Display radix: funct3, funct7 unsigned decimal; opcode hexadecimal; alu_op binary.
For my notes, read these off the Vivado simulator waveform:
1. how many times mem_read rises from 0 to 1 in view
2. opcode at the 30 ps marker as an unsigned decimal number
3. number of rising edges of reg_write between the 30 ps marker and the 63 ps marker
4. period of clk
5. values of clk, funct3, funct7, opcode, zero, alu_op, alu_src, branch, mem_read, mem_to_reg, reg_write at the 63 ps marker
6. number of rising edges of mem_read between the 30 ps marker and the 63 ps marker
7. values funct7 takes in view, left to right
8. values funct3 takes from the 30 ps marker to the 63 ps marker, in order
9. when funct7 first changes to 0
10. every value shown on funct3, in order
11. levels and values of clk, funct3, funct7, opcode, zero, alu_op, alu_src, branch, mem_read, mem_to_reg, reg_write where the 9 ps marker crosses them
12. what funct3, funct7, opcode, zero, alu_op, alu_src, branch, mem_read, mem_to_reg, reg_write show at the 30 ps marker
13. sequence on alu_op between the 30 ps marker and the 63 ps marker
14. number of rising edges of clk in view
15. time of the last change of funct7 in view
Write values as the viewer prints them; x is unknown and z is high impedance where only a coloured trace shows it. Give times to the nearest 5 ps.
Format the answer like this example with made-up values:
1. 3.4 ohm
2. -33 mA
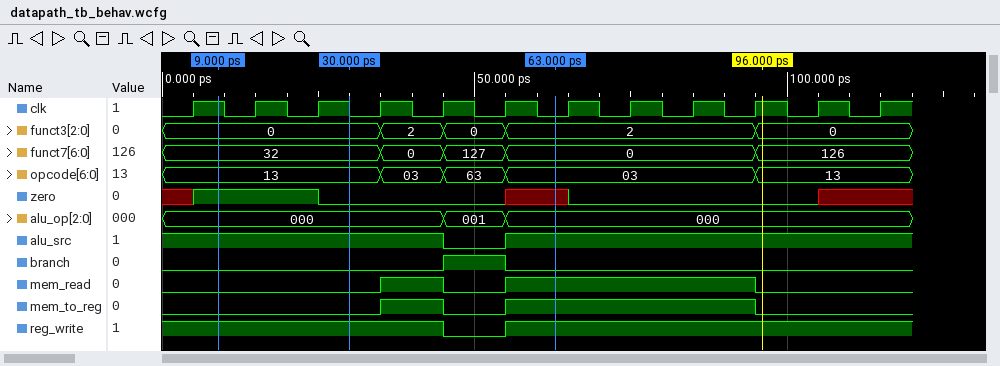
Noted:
1. 2
2. 19
3. 1
4. 10 ps
5. clk=0, funct3=2, funct7=0, opcode=03, zero=x, alu_op=000, alu_src=1, branch=0, mem_read=1, mem_to_reg=1, reg_write=1
6. 2
7. 32, 0, 127, 0, 126
8. 0, 2, 0, 2
9. 35 ps
10. 0, 2, 0, 2, 0
11. clk=1, funct3=0, funct7=32, opcode=13, zero=1, alu_op=000, alu_src=1, branch=0, mem_read=0, mem_to_reg=0, reg_write=1
12. funct3=0, funct7=32, opcode=13, zero=0, alu_op=000, alu_src=1, branch=0, mem_read=0, mem_to_reg=0, reg_write=1
13. 000, 001, 000
14. 12
15. 95 ps
